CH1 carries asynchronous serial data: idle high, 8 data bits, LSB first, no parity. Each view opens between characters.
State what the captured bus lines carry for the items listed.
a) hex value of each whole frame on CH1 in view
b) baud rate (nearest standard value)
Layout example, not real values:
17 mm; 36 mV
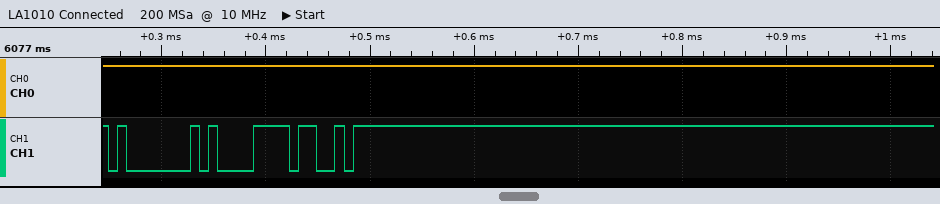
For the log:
01, E1, D3; 115200 baud
